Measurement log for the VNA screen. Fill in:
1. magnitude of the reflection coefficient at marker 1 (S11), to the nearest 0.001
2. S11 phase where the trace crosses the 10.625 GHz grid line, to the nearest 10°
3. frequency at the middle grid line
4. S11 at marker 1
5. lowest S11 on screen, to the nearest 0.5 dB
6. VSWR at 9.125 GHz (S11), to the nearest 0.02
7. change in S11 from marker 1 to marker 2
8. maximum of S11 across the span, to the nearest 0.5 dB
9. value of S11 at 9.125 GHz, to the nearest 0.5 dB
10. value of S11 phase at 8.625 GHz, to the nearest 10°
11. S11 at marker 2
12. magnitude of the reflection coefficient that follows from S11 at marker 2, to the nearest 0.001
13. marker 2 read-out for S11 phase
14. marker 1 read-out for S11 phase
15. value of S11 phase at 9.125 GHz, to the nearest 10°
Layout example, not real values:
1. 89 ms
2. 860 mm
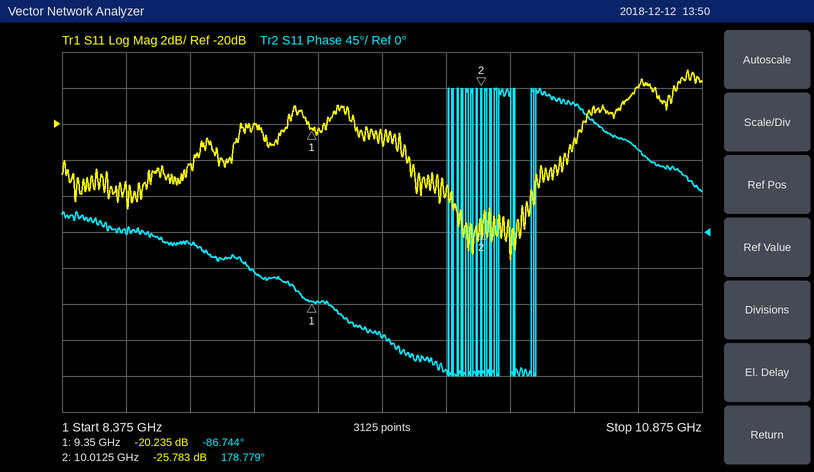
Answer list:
1. 0.097
2. 100°
3. 9.625 GHz
4. -20.235 dB
5. -27.5 dB
6. 1.22
7. -5.548 dB
8. -17.0 dB
9. -20.0 dB
10. 0°
11. -25.783 dB
12. 0.051
13. 178.779°
14. -86.744°
15. -50°
